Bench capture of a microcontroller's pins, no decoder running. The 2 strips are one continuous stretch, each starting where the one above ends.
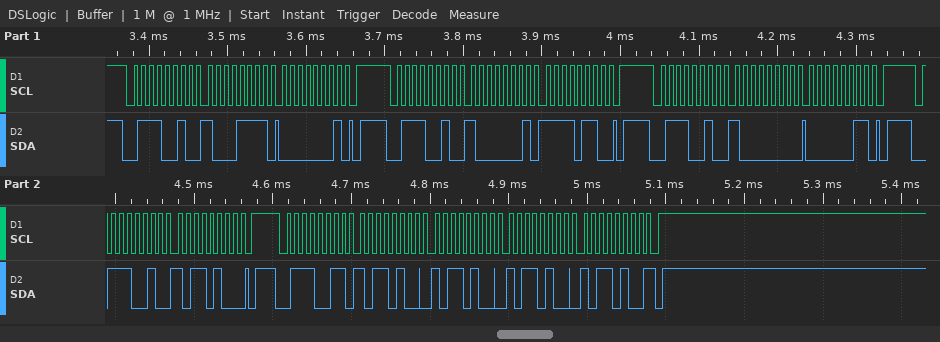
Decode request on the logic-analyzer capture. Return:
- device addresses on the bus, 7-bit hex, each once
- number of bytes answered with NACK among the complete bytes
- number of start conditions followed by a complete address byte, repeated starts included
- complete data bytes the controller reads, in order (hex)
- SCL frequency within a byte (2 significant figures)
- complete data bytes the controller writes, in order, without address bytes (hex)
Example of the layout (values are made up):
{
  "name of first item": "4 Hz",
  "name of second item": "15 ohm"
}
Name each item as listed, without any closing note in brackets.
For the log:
{
  "device addresses on the bus, 7-bit hex, each once": "0x39",
  "number of bytes answered with NACK among the complete bytes": "1",
  "number of start conditions followed by a complete address byte, repeated starts included": "5",
  "complete data bytes the controller reads, in order": "B4 B4 B4 B4",
  "SCL frequency within a byte": "100 kHz",
  "complete data bytes the controller writes, in order, without address bytes": "8F 01 81 F6 80 03 B4"
}
